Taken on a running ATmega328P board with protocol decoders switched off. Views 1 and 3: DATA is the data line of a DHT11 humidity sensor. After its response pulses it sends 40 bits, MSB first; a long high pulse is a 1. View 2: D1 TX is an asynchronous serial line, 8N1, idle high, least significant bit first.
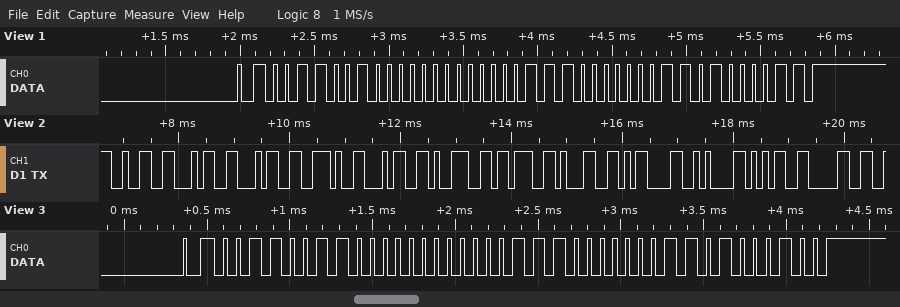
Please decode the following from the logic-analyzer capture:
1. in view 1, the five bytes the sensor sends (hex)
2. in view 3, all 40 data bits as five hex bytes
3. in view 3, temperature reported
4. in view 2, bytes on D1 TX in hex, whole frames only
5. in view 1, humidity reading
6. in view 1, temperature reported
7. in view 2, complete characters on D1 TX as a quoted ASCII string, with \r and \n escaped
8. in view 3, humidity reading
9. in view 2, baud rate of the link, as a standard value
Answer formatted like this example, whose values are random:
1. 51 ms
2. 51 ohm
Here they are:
1. 32 00 0E 03 43
2. 33 00 0E 03 44
3. 14.3 °C
4. 32 34 34 2E 34 39 3B 31 0D 0A 35 30
5. 50 %
6. 14.3 °C
7. "244.49;1\r\n50"
8. 51 %
9. 9600 baud
